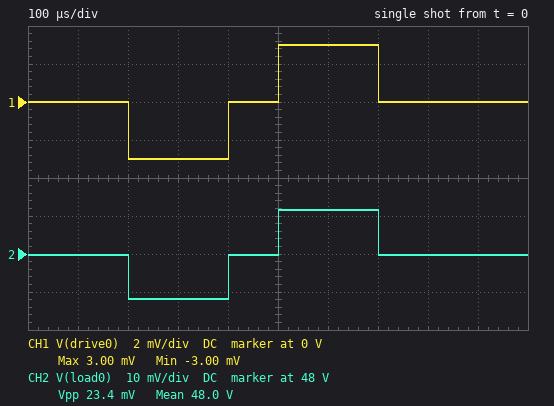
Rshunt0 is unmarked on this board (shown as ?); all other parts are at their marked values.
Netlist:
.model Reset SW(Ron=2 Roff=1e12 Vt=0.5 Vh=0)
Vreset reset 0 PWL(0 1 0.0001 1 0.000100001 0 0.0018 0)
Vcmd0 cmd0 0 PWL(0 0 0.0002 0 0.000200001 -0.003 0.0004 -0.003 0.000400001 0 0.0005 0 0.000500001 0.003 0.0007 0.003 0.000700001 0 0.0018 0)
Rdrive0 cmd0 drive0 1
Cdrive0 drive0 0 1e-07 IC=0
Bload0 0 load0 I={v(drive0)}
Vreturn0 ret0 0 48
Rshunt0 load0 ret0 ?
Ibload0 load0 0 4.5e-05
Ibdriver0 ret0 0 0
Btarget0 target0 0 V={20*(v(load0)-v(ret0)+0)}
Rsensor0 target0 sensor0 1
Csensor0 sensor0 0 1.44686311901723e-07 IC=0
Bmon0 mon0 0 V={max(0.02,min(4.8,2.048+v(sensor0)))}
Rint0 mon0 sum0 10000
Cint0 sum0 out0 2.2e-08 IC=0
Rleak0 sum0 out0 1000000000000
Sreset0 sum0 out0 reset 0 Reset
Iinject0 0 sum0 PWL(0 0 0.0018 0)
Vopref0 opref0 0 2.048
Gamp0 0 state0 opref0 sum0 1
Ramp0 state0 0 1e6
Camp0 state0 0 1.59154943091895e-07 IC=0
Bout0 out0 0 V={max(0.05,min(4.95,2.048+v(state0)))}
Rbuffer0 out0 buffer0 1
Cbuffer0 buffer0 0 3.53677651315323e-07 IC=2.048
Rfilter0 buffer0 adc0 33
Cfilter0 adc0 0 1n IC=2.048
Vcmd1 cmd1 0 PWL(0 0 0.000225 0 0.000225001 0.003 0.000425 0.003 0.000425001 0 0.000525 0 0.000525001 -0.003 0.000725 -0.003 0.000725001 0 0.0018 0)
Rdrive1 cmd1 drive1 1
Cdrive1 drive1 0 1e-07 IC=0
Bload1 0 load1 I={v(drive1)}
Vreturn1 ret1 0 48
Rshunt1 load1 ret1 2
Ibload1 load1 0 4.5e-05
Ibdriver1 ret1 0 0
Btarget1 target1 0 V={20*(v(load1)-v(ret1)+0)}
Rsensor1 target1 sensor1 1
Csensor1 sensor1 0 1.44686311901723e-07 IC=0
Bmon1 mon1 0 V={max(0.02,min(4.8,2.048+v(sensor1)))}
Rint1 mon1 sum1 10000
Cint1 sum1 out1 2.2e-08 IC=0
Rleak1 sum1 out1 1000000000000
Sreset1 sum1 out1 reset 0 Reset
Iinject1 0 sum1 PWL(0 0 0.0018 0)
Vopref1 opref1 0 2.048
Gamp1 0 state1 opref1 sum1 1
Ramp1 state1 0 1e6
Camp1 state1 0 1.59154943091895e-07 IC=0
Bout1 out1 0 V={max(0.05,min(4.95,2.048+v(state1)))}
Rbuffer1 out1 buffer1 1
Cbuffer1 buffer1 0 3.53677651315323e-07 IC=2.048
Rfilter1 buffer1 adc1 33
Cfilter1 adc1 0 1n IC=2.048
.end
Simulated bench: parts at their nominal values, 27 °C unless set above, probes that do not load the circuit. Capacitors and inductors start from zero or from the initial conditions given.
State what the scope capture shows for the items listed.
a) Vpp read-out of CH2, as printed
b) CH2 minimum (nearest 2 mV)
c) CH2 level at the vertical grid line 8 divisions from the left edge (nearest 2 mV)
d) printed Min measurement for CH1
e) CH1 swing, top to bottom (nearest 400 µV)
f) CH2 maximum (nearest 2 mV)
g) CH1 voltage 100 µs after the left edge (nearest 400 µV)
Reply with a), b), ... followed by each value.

a) 23.4 mV
b) 47.988 V
c) 48.000 V
d) -3.00 mV
e) 6.0 mV
f) 48.012 V
g) 0 V
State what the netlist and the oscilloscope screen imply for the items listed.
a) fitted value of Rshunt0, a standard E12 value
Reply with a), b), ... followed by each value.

a) 3.9 Ω
